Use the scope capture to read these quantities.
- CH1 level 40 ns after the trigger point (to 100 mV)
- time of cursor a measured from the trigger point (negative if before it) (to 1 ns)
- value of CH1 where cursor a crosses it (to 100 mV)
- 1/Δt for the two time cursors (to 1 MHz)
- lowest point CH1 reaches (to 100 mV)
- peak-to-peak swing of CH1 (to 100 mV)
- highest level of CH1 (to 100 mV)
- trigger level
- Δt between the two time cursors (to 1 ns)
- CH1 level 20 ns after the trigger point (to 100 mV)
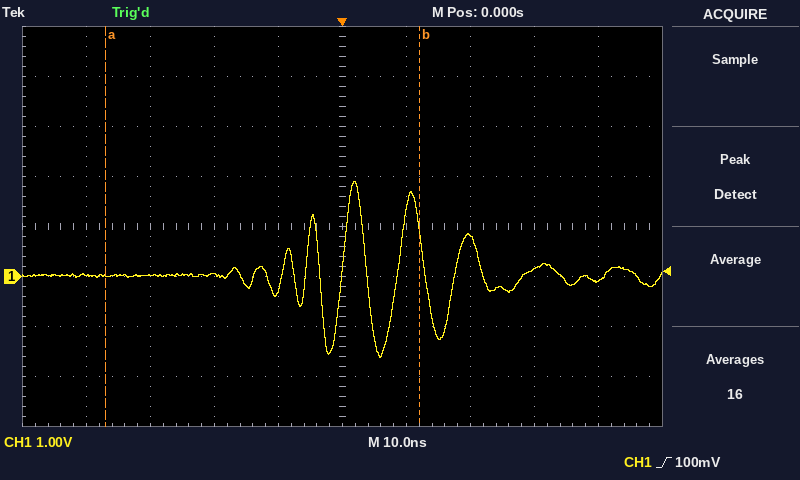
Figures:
-100 mV
-37 ns
0.0 V
20 MHz
-1.6 V
3.5 V
1.9 V
100 mV
49 ns
800 mV
